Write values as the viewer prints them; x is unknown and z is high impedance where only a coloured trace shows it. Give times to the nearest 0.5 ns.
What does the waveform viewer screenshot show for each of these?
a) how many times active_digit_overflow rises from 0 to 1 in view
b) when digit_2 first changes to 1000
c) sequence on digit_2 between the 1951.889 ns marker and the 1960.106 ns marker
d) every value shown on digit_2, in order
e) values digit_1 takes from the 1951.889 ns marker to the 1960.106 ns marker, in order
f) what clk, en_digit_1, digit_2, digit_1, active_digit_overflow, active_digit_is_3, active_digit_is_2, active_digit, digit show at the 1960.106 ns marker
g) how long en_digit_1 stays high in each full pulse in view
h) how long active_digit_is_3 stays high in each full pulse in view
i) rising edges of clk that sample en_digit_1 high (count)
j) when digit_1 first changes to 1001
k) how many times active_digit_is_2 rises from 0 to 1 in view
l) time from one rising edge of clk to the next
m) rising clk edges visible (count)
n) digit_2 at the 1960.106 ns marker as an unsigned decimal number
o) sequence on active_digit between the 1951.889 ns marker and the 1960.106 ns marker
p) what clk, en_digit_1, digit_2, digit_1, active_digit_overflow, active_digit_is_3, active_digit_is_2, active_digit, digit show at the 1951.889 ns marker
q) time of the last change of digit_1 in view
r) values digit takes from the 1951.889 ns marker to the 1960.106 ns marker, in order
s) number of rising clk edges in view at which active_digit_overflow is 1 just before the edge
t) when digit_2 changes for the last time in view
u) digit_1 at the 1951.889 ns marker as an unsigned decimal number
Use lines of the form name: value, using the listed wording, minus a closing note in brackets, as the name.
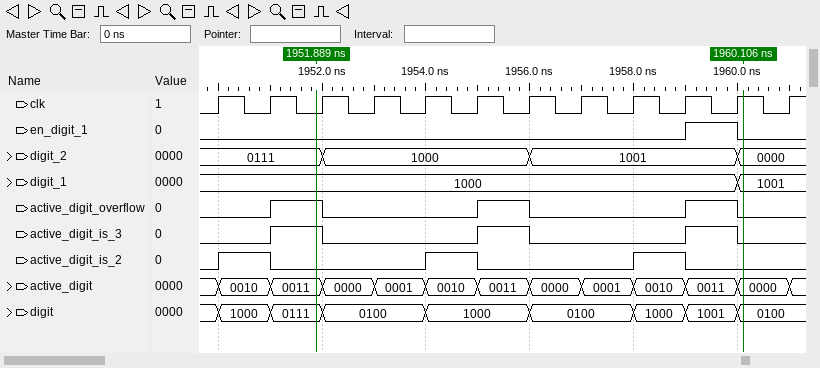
how many times active_digit_overflow rises from 0 to 1 in view: 3
when digit_2 first changes to 1000: 1952 ns
sequence on digit_2 between the 1951.889 ns marker and the 1960.106 ns marker: 0111, 1000, 1001, 0000
every value shown on digit_2, in order: 0111, 1000, 1001, 0000
values digit_1 takes from the 1951.889 ns marker to the 1960.106 ns marker, in order: 1000, 1001
what clk, en_digit_1, digit_2, digit_1, active_digit_overflow, active_digit_is_3, active_digit_is_2, active_digit, digit show at the 1960.106 ns marker: clk=1, en_digit_1=0, digit_2=0000, digit_1=1001, active_digit_overflow=0, active_digit_is_3=0, active_digit_is_2=0, active_digit=0000, digit=0100
how long en_digit_1 stays high in each full pulse in view: 1 ns
how long active_digit_is_3 stays high in each full pulse in view: 1 ns, 1 ns, 1 ns
rising edges of clk that sample en_digit_1 high: 1
when digit_1 first changes to 1001: 1960 ns
how many times active_digit_is_2 rises from 0 to 1 in view: 3
time from one rising edge of clk to the next: 1 ns
rising clk edges visible: 12
digit_2 at the 1960.106 ns marker as an unsigned decimal number: 0
sequence on active_digit between the 1951.889 ns marker and the 1960.106 ns marker: 0011, 0000, 0001, 0010, 0011, 0000, 0001, 0010, 0011, 0000
what clk, en_digit_1, digit_2, digit_1, active_digit_overflow, active_digit_is_3, active_digit_is_2, active_digit, digit show at the 1951.889 ns marker: clk=0, en_digit_1=0, digit_2=0111, digit_1=1000, active_digit_overflow=1, active_digit_is_3=1, active_digit_is_2=0, active_digit=0011, digit=0111
time of the last change of digit_1 in view: 1960 ns
values digit takes from the 1951.889 ns marker to the 1960.106 ns marker, in order: 0111, 0100, 1000, 0100, 1000, 1001, 0100
number of rising clk edges in view at which active_digit_overflow is 1 just before the edge: 3
when digit_2 changes for the last time in view: 1960 ns
digit_1 at the 1951.889 ns marker as an unsigned decimal number: 8
